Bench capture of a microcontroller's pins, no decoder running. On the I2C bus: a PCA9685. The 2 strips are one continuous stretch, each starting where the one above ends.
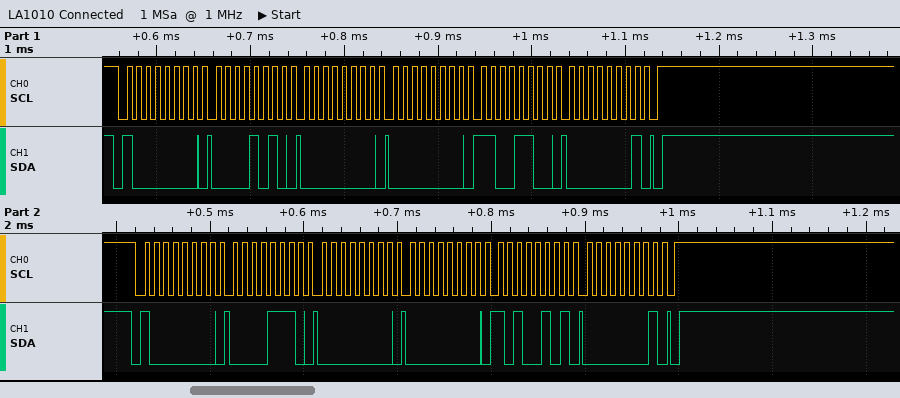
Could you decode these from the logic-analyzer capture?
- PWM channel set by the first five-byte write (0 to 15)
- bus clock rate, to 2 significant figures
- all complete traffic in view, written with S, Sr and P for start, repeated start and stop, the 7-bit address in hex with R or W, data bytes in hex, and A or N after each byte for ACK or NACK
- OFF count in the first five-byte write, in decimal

1
100 kHz
S 40W A 0A A 00 A 00 A CC A 01 A P S 40W A 0E A 00 A 00 A A5 A 01 A P
460
